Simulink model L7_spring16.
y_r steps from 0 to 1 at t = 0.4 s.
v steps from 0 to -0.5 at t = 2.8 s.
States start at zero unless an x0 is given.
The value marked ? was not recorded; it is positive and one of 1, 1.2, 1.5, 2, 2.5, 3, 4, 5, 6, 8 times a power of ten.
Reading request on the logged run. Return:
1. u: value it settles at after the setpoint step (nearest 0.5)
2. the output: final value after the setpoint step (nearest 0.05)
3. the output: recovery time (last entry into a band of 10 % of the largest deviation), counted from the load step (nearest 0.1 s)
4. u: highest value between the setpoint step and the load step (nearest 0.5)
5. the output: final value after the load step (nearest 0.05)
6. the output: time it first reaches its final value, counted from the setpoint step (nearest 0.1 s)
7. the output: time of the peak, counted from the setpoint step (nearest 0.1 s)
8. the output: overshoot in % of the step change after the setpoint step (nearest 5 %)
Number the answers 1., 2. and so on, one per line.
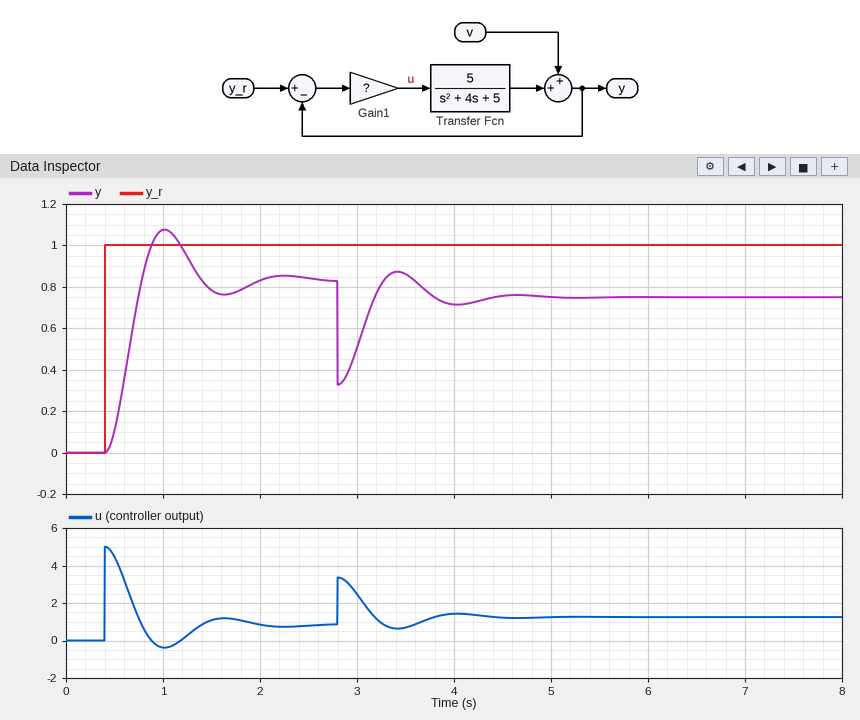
1. 1.0
2. 0.85
3. 0.9 s
4. 5.0
5. 0.75
6. 0.4 s
7. 0.6 s
8. 30 %
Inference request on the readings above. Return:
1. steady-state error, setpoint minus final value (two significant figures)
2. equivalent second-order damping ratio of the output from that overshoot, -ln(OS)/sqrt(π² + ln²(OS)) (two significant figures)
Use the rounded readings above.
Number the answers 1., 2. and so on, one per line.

1. 0.15
2. 0.36
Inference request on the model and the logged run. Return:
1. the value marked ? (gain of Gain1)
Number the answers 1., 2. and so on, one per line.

1. 5
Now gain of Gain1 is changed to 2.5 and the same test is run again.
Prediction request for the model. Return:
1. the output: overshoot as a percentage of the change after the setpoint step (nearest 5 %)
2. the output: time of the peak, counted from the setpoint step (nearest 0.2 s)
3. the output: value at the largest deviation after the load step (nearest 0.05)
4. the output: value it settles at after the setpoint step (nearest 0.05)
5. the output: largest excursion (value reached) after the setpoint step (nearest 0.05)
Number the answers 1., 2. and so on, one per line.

1. 20 %
2. 0.8 s
3. 0.20
4. 0.70
5. 0.85
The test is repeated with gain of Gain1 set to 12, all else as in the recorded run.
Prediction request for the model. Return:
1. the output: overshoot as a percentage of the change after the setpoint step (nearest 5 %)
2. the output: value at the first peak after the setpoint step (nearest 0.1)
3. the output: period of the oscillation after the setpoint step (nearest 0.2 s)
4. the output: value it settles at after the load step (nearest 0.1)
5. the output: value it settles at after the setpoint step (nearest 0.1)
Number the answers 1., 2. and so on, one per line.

1. 45 %
2. 1.3
3. 0.8 s
4. 0.9
5. 0.9
